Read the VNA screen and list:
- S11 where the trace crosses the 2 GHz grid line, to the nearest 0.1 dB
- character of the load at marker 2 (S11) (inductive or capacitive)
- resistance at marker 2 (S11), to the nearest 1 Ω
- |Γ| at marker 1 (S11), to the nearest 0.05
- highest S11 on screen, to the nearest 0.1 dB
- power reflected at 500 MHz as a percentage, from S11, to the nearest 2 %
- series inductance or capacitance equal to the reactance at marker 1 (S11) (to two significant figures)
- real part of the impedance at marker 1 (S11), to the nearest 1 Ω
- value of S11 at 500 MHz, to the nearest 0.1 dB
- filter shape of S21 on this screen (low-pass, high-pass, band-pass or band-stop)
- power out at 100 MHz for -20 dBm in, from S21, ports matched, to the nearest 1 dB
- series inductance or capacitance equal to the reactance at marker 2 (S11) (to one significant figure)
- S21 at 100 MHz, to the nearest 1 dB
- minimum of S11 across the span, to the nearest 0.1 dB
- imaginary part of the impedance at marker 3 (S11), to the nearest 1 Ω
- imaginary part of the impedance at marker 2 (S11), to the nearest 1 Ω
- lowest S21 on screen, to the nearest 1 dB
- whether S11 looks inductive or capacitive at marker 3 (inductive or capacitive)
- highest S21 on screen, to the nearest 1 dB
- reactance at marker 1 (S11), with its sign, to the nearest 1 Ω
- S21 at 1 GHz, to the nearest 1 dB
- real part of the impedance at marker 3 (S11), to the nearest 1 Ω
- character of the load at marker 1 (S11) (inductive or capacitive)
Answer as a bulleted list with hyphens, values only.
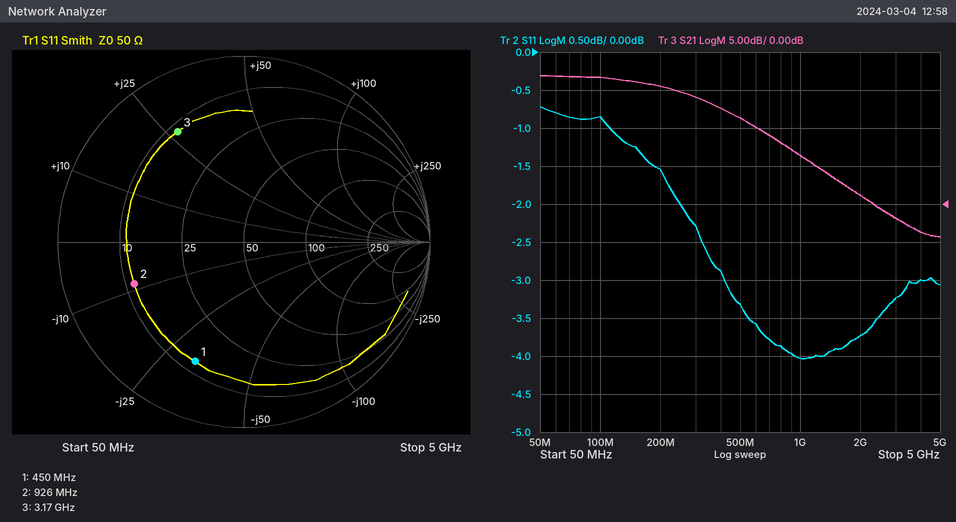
- -3.7 dB
- capacitive
- 12 Ω
- 0.70
- -0.7 dB
- 46 %
- 11 pF
- 13 Ω
- -3.3 dB
- low-pass
- -3 dBm
- 20 pF
- 17 dB
- -4.0 dB
- +27 Ω
- -9 Ω
- -4 dB
- inductive
- 17 dB
- -32 Ω
- 6 dB
- 12 Ω
- capacitive
